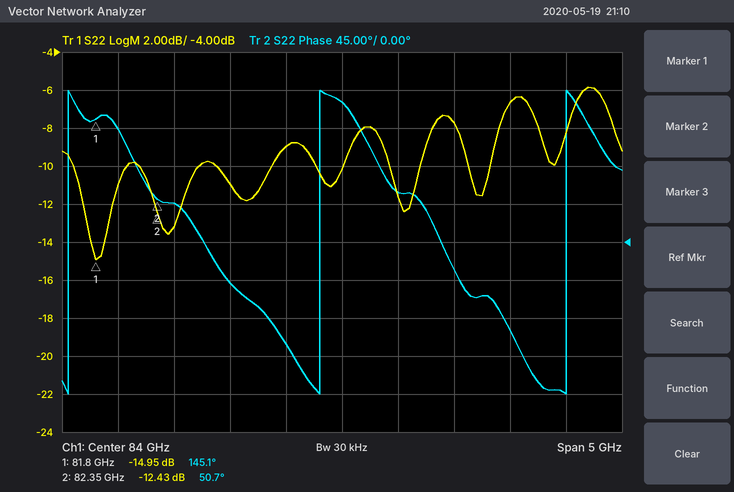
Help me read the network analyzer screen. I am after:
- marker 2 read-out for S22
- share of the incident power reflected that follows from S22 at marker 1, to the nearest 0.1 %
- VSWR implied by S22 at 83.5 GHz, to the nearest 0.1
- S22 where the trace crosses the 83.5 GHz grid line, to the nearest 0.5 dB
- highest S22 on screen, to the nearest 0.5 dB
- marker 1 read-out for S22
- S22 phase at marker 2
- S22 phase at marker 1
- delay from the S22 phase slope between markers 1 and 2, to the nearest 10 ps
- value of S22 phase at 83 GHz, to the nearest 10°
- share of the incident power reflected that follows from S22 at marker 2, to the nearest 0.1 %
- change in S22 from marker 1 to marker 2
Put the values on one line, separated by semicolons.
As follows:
-12.43 dB; 3.2 %; 2.1; -9.0 dB; -6.0 dB; -14.95 dB; 50.7°; 145.1°; 480 ps; -50°; 5.7 %; 2.52 dB
